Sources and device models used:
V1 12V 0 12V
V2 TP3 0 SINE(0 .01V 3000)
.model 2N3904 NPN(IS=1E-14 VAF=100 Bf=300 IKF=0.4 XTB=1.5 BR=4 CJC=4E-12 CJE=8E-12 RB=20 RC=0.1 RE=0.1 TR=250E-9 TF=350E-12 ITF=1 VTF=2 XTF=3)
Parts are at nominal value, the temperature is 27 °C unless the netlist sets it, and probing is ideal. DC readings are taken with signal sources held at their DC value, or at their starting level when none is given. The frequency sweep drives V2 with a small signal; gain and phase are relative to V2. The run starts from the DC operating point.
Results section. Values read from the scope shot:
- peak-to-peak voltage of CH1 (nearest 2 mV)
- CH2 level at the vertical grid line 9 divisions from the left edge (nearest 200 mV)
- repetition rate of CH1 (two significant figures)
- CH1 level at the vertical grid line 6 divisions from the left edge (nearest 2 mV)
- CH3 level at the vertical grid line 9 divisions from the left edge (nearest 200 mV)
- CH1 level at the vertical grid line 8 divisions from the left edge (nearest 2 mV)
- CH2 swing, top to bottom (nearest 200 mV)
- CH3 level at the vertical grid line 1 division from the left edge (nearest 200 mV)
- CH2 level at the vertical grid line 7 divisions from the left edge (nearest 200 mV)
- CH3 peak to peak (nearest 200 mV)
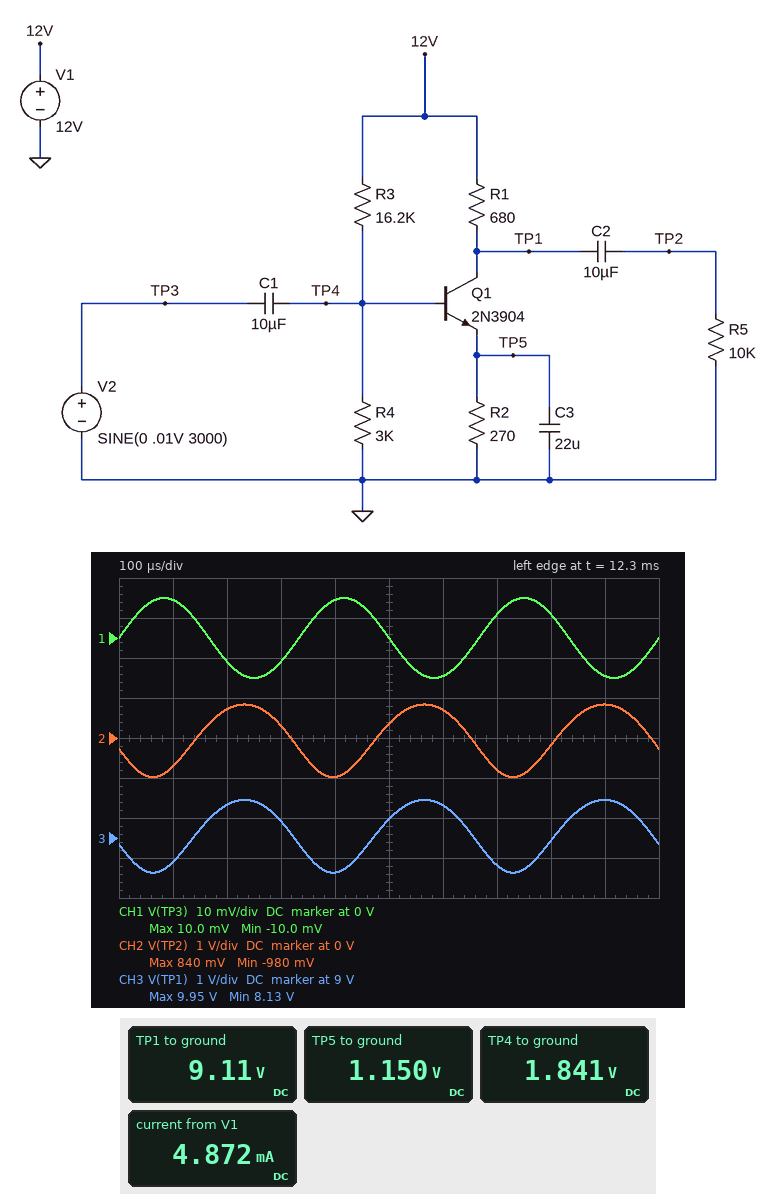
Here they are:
20 mV
800 mV
3.0 kHz
-10 mV
10.0 V
6 mV
1.8 V
8.4 V
-800 mV
1.8 V
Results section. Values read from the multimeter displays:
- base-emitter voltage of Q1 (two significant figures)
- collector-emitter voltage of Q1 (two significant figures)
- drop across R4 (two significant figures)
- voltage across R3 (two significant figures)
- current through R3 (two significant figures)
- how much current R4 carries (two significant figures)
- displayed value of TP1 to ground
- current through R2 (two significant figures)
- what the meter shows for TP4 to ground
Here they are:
690 mV
8.0 V
1.8 V
10 V
630 µA
610 µA
9.11 V
4.3 mA
1.841 V
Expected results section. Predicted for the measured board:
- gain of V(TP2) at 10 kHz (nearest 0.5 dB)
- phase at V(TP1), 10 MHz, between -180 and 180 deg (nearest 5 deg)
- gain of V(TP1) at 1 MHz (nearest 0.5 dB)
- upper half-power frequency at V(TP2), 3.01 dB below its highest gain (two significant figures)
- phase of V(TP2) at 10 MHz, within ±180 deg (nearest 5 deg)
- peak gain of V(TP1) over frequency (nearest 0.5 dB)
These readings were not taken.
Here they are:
40.0 dB
160 deg
40.0 dB
27 MHz
160 deg
40.0 dB
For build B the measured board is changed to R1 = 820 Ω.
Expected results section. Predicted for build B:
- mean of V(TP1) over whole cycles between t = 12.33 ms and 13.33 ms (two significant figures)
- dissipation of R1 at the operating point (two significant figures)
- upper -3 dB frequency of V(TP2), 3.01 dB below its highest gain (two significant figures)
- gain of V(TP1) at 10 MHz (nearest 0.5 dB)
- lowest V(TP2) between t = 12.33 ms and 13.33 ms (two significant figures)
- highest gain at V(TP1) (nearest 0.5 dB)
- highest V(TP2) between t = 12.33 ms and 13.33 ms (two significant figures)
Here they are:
8.5 V
15 mW
23 MHz
40.5 dB
-1.2 V
41.5 dB
990 mV
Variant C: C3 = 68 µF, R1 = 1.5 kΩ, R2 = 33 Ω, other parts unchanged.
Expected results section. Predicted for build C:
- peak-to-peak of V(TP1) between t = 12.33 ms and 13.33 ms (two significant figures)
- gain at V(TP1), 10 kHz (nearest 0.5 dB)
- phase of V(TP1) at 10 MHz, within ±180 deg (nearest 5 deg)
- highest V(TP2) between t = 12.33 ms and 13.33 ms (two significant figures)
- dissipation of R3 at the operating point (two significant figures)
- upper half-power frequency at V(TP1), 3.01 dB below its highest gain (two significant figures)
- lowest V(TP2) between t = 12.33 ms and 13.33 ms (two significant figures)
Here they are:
63 mV
6.0 dB
20 deg
49 mV
7.5 mW
240 kHz
-14 mV
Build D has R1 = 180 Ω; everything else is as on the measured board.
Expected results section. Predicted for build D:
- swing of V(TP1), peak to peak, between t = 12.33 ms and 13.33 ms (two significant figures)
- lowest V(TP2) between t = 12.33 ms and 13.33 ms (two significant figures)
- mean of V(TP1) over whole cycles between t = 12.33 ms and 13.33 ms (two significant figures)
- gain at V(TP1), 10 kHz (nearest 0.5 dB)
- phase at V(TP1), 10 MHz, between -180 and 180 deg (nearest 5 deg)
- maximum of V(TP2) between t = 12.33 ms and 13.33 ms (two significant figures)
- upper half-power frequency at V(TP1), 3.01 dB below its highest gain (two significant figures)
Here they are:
510 mV
-280 mV
11 V
29.0 dB
170 deg
240 mV
64 MHz
